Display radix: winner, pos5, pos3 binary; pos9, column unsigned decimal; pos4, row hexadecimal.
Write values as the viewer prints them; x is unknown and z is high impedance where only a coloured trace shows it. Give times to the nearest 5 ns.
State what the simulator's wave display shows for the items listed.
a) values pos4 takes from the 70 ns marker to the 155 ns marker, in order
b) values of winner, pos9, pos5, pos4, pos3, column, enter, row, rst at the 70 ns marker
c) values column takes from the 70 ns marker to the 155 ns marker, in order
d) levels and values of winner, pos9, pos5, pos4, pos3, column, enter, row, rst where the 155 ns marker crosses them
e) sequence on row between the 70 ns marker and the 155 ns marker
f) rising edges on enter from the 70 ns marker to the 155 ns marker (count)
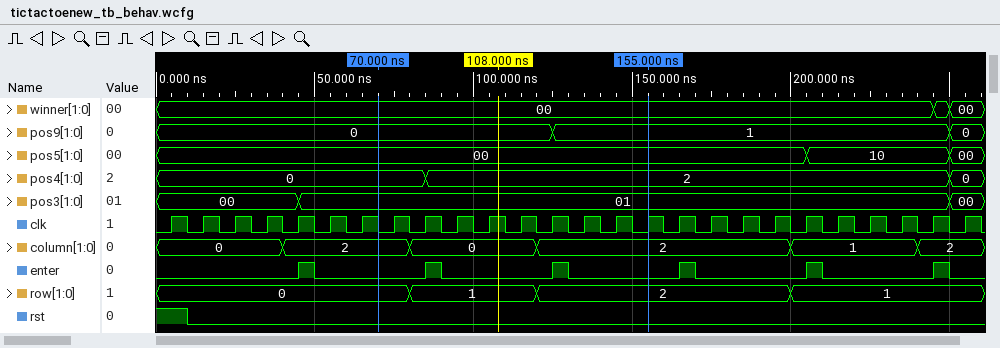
0, 2
winner=00, pos9=0, pos5=00, pos4=0, pos3=01, column=2, enter=0, row=0, rst=0
2, 0, 2
winner=00, pos9=1, pos5=00, pos4=2, pos3=01, column=2, enter=0, row=2, rst=0
0, 1, 2
2
